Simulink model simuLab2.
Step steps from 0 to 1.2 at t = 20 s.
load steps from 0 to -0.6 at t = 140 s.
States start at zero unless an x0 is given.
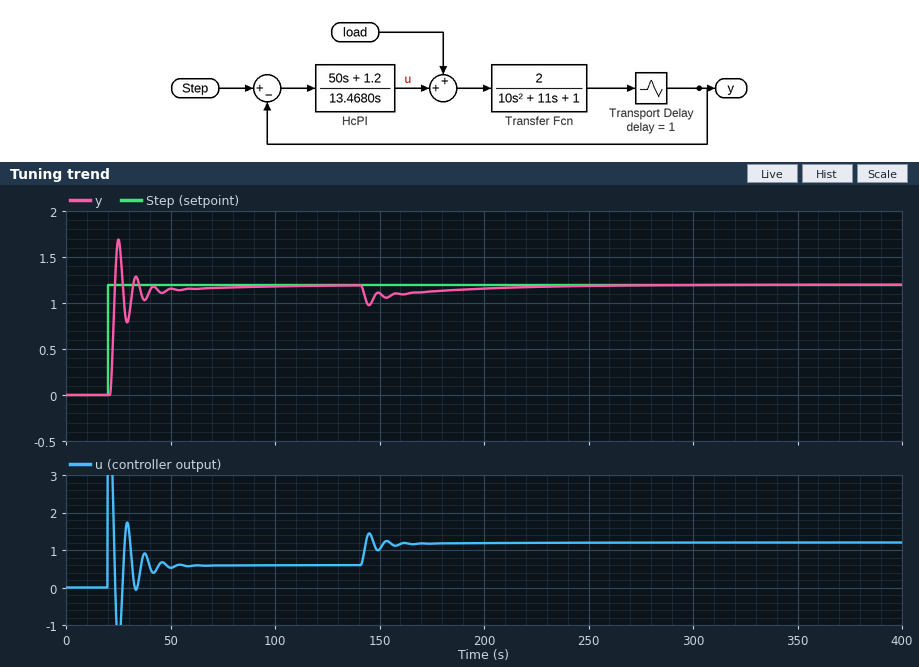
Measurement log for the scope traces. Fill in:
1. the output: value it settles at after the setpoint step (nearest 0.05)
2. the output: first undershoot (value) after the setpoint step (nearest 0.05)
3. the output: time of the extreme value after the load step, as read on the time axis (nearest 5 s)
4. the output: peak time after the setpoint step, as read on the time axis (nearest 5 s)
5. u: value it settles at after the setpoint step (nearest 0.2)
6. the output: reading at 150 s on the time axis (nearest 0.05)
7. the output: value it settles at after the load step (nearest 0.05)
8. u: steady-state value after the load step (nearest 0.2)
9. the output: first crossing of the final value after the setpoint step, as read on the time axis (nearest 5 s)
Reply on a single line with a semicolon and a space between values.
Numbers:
1.20; 0.80; 145 s; 25 s; 0.6; 1.10; 1.20; 1.2; 25 s
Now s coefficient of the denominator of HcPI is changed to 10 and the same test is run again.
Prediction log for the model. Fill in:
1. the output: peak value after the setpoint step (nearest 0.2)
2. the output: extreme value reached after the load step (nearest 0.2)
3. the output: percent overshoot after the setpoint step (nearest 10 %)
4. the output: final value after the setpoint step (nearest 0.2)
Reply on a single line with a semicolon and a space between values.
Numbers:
2.0; 1.0; 70 %; 1.2
